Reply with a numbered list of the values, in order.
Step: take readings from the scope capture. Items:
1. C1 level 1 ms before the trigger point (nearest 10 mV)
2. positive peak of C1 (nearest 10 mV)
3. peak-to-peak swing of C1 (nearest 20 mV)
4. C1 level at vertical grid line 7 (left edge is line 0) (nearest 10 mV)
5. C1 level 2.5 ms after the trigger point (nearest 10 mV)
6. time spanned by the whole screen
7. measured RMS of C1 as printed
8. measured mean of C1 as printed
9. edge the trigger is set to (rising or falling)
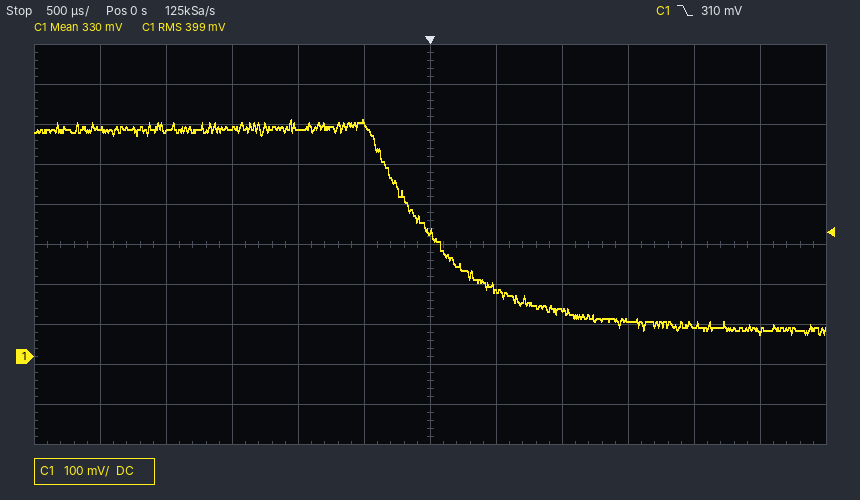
1. 570 mV
2. 590 mV
3. 540 mV
4. 170 mV
5. 60 mV
6. 6 ms
7. 399 mV
8. 330 mV
9. falling
